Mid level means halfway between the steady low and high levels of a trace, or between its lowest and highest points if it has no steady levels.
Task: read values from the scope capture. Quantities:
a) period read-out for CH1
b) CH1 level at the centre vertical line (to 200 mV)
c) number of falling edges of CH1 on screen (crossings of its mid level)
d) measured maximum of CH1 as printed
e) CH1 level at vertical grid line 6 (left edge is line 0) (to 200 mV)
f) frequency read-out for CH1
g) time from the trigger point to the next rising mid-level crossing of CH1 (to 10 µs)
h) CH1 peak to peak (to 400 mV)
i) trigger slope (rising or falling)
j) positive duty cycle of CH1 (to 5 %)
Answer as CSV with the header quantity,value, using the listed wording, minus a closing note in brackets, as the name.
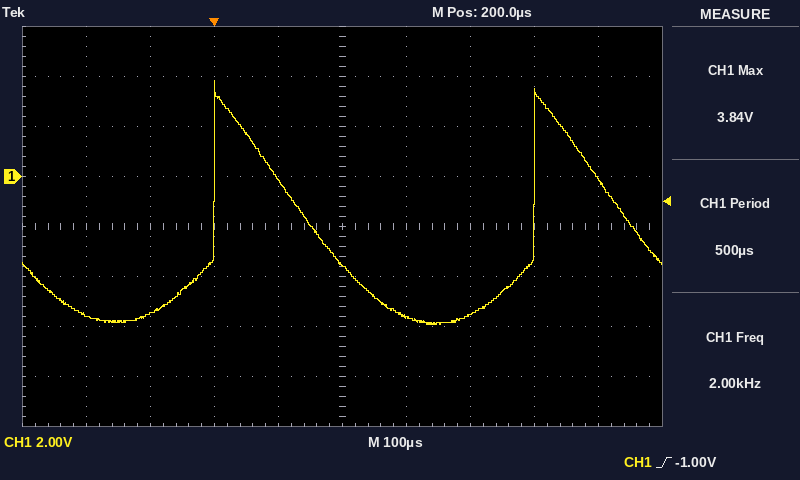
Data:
quantity,value
period read-out for CH1,500 µs
CH1 level at the centre vertical line,-3.6 V
number of falling edges of CH1 on screen,2
measured maximum of CH1 as printed,3.84 V
CH1 level at vertical grid line 6 (left edge is line 0),-5.6 V
frequency read-out for CH1,2.00 kHz
time from the trigger point to the next rising mid-level crossing of CH1,500 µs
CH1 peak to peak,9.6 V
trigger slope,rising
positive duty cycle of CH1,25 %
